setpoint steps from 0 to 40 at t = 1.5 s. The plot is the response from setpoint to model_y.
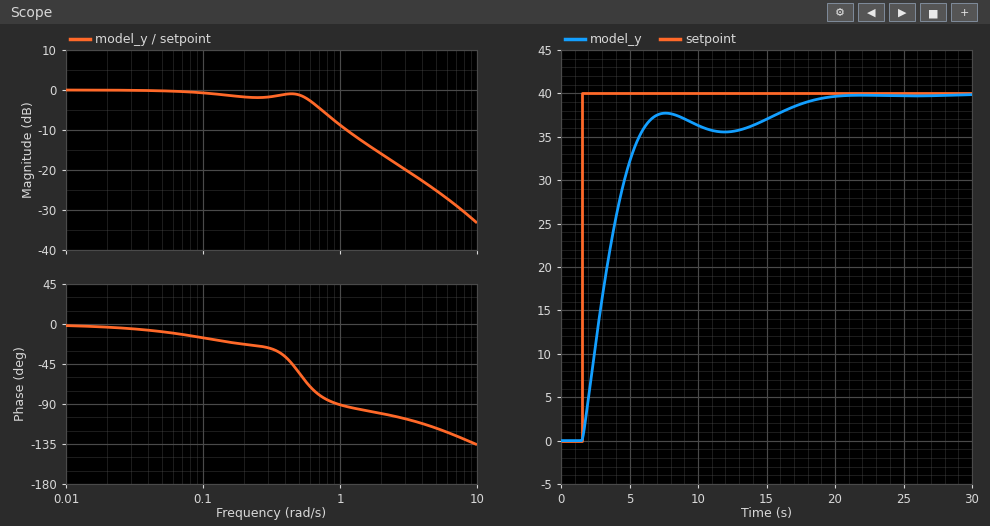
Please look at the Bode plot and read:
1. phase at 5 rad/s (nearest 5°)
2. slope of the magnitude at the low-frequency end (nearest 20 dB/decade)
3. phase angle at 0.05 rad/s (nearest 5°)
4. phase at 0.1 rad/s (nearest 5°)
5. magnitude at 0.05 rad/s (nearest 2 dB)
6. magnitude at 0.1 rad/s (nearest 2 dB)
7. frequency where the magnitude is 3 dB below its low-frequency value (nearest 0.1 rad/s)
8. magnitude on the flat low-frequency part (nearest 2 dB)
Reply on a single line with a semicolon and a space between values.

-115°; 0 dB/decade; -10°; -15°; 0 dB; 0 dB; 0.6 rad/s; 0 dB
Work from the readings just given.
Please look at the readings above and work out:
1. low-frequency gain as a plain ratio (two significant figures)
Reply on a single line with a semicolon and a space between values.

1.0
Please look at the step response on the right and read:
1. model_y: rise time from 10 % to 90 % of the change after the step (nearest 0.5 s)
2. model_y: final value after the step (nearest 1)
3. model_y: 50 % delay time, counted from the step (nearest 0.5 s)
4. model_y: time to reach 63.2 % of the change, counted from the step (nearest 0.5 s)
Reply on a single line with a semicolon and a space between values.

4.0 s; 40; 2.0 s; 2.5 s
